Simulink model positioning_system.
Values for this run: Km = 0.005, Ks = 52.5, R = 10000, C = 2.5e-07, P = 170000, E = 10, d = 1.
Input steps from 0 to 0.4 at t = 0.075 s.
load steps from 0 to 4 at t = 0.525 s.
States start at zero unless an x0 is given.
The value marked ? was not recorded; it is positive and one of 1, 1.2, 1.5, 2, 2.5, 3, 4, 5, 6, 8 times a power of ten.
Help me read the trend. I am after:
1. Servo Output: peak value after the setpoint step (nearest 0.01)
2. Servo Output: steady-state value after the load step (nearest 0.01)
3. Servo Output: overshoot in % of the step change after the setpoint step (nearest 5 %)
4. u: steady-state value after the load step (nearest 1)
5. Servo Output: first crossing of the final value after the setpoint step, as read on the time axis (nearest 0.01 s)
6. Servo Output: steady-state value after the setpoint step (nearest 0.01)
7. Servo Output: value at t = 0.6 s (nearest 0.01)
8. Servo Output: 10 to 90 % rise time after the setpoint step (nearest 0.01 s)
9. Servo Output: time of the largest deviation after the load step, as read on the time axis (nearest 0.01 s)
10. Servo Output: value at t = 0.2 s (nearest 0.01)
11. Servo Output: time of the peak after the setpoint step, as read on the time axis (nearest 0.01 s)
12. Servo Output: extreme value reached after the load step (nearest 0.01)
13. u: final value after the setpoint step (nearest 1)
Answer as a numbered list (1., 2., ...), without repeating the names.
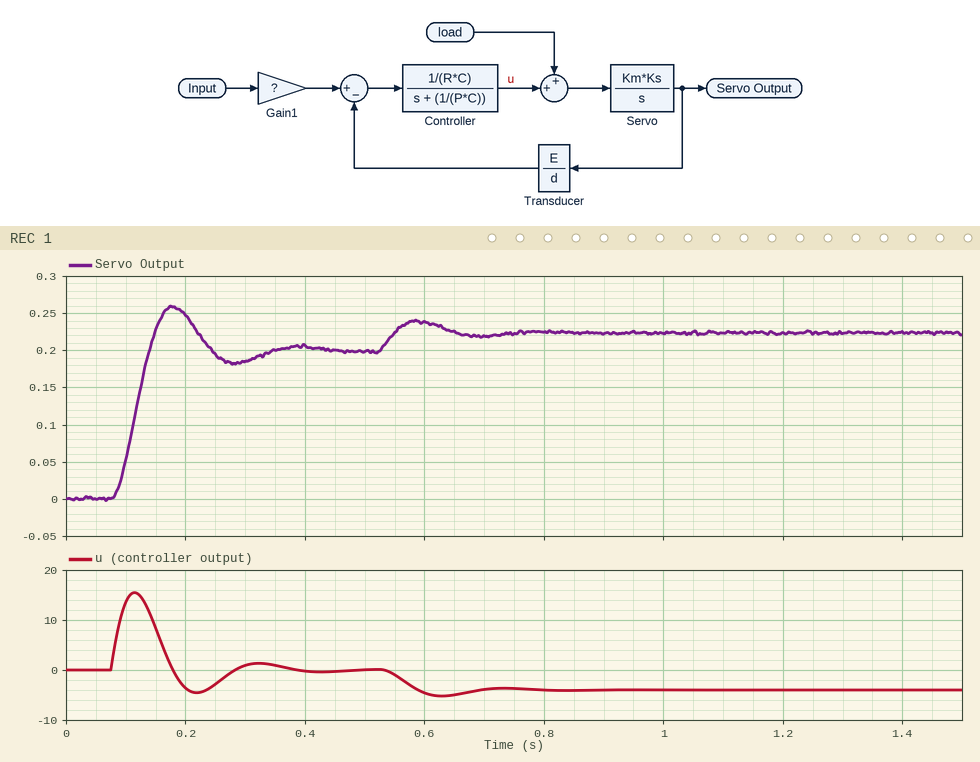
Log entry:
1. 0.26
2. 0.22
3. 30 %
4. -4
5. 0.14 s
6. 0.20
7. 0.24
8. 0.04 s
9. 0.59 s
10. 0.25
11. 0.18 s
12. 0.24
13. 0
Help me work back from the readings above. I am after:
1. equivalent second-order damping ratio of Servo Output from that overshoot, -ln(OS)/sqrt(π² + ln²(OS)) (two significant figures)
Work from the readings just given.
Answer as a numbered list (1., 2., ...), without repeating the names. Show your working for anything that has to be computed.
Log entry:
1. ln(0.3) = -1.204; 1.204 / sqrt(9.870 + 1.450) = 0.36
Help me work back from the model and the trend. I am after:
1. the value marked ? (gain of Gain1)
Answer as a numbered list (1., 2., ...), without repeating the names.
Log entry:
1. 5
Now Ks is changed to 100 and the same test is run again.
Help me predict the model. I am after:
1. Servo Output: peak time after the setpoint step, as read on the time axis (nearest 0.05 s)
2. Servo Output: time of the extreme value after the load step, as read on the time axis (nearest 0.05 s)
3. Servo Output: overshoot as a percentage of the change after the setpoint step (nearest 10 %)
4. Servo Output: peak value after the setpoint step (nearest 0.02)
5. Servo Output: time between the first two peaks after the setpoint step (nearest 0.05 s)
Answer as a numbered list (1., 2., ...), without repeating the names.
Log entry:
1. 0.15 s
2. 0.55 s
3. 40 %
4. 0.28
5. 0.15 s
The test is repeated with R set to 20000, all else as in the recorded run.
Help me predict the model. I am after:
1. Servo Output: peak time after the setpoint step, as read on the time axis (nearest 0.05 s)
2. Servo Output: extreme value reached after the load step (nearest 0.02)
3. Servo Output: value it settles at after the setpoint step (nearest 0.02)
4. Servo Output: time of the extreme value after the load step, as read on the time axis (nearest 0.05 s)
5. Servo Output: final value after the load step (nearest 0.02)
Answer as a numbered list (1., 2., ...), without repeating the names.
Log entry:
1. 0.25 s
2. 0.26
3. 0.20
4. 0.65 s
5. 0.24
